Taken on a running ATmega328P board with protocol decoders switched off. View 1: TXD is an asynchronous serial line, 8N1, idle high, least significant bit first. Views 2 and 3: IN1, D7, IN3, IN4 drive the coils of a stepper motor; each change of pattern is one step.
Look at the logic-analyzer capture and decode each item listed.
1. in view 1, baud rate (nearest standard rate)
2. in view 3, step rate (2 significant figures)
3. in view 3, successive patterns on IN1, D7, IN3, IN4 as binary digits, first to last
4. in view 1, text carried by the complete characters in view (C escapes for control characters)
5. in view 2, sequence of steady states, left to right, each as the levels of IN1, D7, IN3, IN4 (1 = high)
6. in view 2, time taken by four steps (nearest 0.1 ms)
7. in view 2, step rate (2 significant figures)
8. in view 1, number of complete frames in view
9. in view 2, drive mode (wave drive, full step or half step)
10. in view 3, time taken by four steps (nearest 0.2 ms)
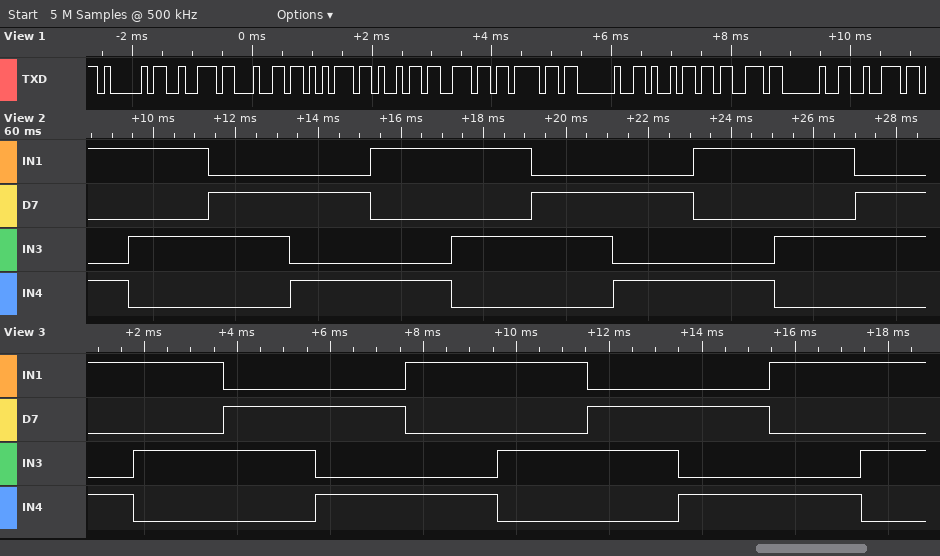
9600 baud
510 steps/s
1001 1010 0110 0101 1001 1010 0110 0101 1001 1010
"Arduino is r"
1001 1010 0110 0101 1001 1010 0110 0101 1001 1010 0110
7.8 ms
510 steps/s
12
full step
7.8 ms
